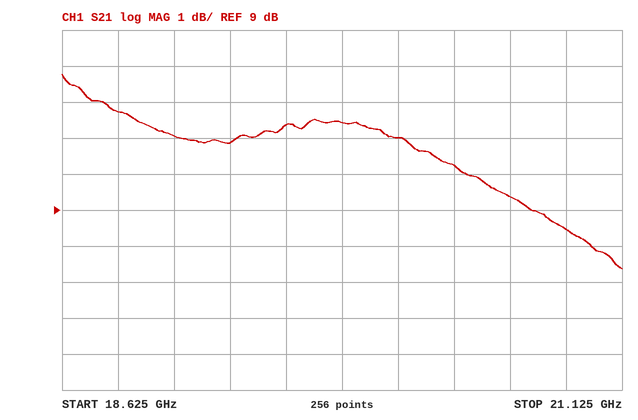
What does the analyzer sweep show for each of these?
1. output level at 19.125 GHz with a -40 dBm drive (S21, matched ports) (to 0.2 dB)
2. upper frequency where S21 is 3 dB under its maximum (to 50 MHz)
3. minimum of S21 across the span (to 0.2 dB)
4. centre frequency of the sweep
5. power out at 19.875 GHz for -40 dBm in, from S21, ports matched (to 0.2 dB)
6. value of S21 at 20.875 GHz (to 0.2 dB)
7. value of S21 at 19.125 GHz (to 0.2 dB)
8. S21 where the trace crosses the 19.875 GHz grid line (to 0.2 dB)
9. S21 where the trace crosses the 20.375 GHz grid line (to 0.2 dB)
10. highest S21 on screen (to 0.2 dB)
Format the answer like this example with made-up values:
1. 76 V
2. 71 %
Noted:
1. -29.0 dBm
2. 20.50 GHz
3. 7.4 dB
4. 19.875 GHz
5. -28.6 dBm
6. 8.4 dB
7. 11.0 dB
8. 11.4 dB
9. 10.2 dB
10. 12.8 dB
